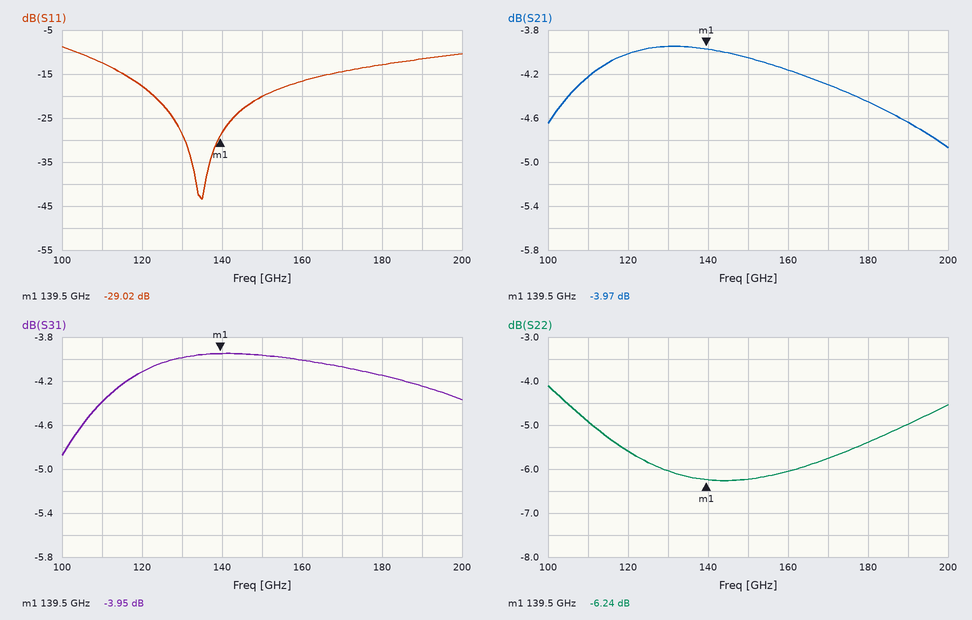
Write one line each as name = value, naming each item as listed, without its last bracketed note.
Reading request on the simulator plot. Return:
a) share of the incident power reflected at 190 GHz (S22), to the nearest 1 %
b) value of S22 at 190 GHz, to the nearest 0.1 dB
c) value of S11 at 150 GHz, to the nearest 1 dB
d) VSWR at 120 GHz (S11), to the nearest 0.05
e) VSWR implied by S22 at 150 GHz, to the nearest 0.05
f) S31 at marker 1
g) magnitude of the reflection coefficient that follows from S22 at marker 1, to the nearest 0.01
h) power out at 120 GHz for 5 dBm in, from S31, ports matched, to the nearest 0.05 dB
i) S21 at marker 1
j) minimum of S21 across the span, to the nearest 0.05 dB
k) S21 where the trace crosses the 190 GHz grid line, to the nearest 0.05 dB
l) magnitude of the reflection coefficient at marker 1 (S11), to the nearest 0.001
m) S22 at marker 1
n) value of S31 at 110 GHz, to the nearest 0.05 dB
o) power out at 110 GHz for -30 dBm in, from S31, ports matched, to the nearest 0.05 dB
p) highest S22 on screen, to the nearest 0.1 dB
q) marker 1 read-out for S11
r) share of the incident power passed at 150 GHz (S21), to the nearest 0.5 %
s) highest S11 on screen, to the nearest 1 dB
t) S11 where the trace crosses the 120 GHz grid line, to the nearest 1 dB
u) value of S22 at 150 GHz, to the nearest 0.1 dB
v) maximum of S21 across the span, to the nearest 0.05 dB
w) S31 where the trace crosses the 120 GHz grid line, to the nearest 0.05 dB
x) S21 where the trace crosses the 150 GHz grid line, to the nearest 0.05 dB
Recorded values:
share of the incident power reflected at 190 GHz (S22), to the nearest 1 % = 32 %
value of S22 at 190 GHz, to the nearest 0.1 dB = -5.0 dB
value of S11 at 150 GHz, to the nearest 1 dB = -20 dB
VSWR at 120 GHz (S11), to the nearest 0.05 = 1.30
VSWR implied by S22 at 150 GHz, to the nearest 0.05 = 2.90
S31 at marker 1 = -3.95 dB
magnitude of the reflection coefficient that follows from S22 at marker 1, to the nearest 0.01 = 0.49
power out at 120 GHz for 5 dBm in, from S31, ports matched, to the nearest 0.05 dB = 0.90 dBm
S21 at marker 1 = -3.97 dB
minimum of S21 across the span, to the nearest 0.05 dB = -4.85 dB
S21 where the trace crosses the 190 GHz grid line, to the nearest 0.05 dB = -4.65 dB
magnitude of the reflection coefficient at marker 1 (S11), to the nearest 0.001 = 0.035
S22 at marker 1 = -6.24 dB
value of S31 at 110 GHz, to the nearest 0.05 dB = -4.40 dB
power out at 110 GHz for -30 dBm in, from S31, ports matched, to the nearest 0.05 dB = -34.40 dBm
highest S22 on screen, to the nearest 0.1 dB = -4.1 dB
marker 1 read-out for S11 = -29.02 dB
share of the incident power passed at 150 GHz (S21), to the nearest 0.5 % = 39.5 %
highest S11 on screen, to the nearest 1 dB = -9 dB
S11 where the trace crosses the 120 GHz grid line, to the nearest 1 dB = -18 dB
value of S22 at 150 GHz, to the nearest 0.1 dB = -6.2 dB
maximum of S21 across the span, to the nearest 0.05 dB = -3.95 dB
S31 where the trace crosses the 120 GHz grid line, to the nearest 0.05 dB = -4.10 dB
S21 where the trace crosses the 150 GHz grid line, to the nearest 0.05 dB = -4.05 dB
